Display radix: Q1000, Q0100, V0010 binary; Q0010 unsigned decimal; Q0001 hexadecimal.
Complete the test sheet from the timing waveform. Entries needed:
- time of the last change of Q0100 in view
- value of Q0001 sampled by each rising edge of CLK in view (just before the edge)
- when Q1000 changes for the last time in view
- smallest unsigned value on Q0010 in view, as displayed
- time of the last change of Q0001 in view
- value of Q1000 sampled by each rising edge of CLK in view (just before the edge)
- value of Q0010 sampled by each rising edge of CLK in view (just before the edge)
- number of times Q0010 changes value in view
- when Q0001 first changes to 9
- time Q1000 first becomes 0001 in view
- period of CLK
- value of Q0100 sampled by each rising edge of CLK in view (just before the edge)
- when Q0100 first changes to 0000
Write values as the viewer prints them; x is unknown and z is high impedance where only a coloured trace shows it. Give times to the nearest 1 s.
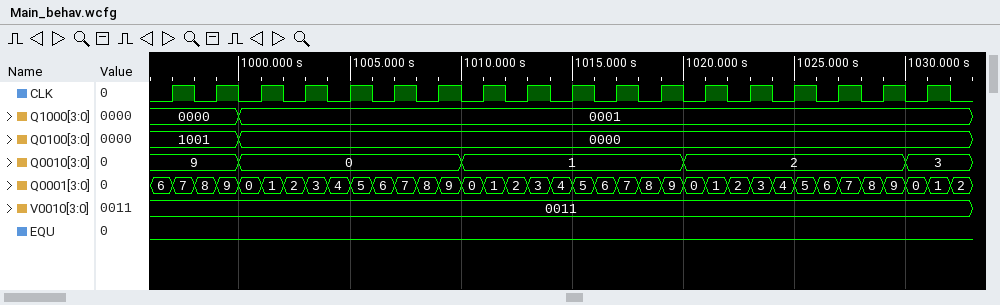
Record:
1000 s
6, 8, 0, 2, 4, 6, 8, 0, 2, 4, 6, 8, 0, 2, 4, 6, 8, 0
1000 s
0
1032 s
0000, 0000, 0001, 0001, 0001, 0001, 0001, 0001, 0001, 0001, 0001, 0001, 0001, 0001, 0001, 0001, 0001, 0001
9, 9, 0, 0, 0, 0, 0, 1, 1, 1, 1, 1, 2, 2, 2, 2, 2, 3
4
999 s
1000 s
2 s
1001, 1001, 0000, 0000, 0000, 0000, 0000, 0000, 0000, 0000, 0000, 0000, 0000, 0000, 0000, 0000, 0000, 0000
1000 s
